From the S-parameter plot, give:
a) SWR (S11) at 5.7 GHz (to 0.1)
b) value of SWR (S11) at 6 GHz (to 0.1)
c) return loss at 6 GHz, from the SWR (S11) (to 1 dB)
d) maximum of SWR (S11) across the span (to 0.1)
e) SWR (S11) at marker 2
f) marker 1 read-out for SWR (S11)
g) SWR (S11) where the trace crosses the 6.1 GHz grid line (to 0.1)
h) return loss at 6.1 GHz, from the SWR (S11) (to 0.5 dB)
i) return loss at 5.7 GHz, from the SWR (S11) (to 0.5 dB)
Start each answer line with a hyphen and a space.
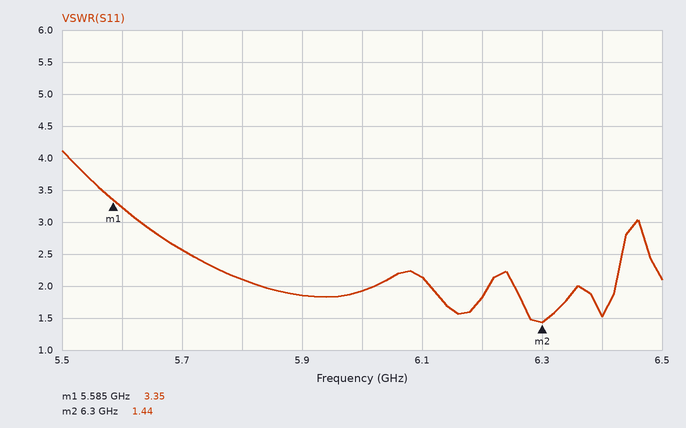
- 2.6
- 1.9
- 10 dB
- 4.1
- 1.44
- 3.35
- 2.1
- 9.0 dB
- 7.0 dB
